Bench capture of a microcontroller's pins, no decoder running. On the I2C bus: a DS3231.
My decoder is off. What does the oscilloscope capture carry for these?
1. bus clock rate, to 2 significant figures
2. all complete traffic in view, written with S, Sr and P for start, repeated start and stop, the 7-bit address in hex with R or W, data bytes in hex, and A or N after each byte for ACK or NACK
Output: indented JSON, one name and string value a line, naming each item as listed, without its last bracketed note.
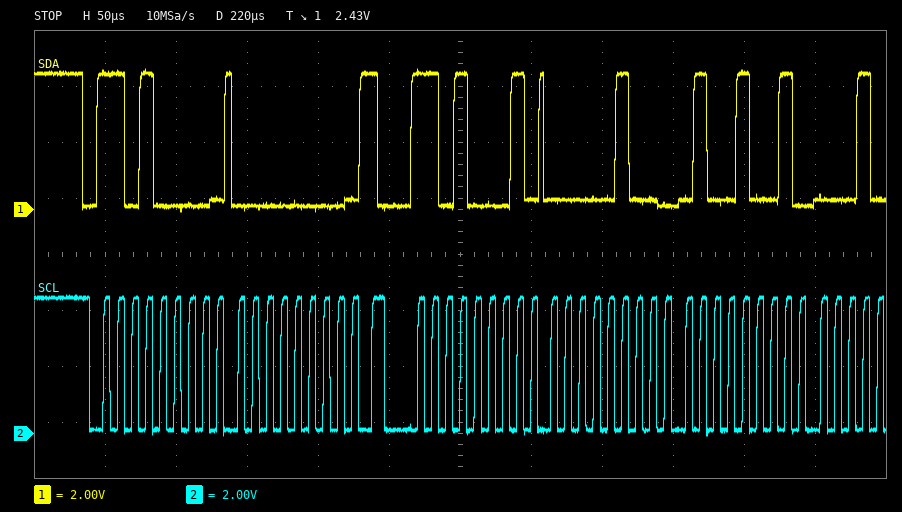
{
  "bus clock rate, to 2 significant figures": "100 kHz",
  "all complete traffic in view, written with S, Sr and P for start, repeated start and stop, the 7-bit address in hex with R or W, data bytes in hex, and A or N after each byte for ACK or NACK": "S 68W A 00 A Sr 68R A 04 A 49 A"
}
